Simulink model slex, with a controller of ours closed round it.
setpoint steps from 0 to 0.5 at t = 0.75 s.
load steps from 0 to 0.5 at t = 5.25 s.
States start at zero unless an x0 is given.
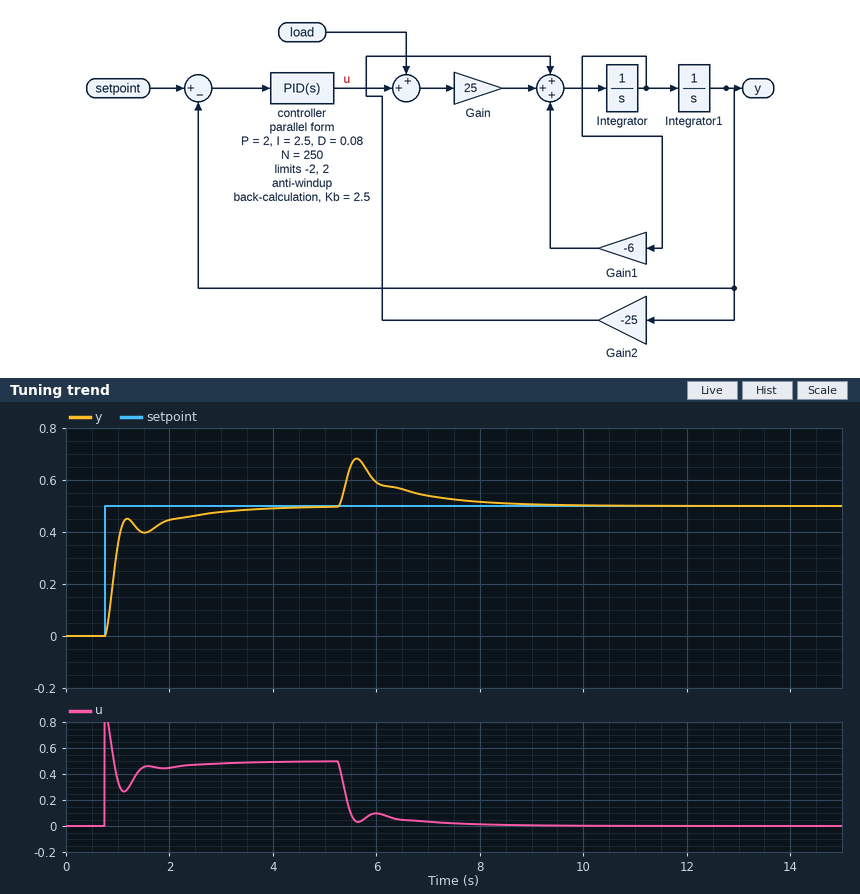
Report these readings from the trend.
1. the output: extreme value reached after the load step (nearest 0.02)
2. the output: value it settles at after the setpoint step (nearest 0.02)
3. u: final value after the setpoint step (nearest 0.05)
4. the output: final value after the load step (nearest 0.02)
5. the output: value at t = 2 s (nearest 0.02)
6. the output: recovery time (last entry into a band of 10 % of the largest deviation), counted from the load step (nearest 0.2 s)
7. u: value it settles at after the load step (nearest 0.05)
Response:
0.68
0.50
0.50
0.50
0.44
2.6 s
0.00
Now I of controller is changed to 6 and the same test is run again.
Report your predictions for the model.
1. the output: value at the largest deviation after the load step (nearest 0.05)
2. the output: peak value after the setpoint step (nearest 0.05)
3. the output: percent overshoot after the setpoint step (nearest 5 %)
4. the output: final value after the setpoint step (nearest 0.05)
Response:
0.65
0.55
10 %
0.50
